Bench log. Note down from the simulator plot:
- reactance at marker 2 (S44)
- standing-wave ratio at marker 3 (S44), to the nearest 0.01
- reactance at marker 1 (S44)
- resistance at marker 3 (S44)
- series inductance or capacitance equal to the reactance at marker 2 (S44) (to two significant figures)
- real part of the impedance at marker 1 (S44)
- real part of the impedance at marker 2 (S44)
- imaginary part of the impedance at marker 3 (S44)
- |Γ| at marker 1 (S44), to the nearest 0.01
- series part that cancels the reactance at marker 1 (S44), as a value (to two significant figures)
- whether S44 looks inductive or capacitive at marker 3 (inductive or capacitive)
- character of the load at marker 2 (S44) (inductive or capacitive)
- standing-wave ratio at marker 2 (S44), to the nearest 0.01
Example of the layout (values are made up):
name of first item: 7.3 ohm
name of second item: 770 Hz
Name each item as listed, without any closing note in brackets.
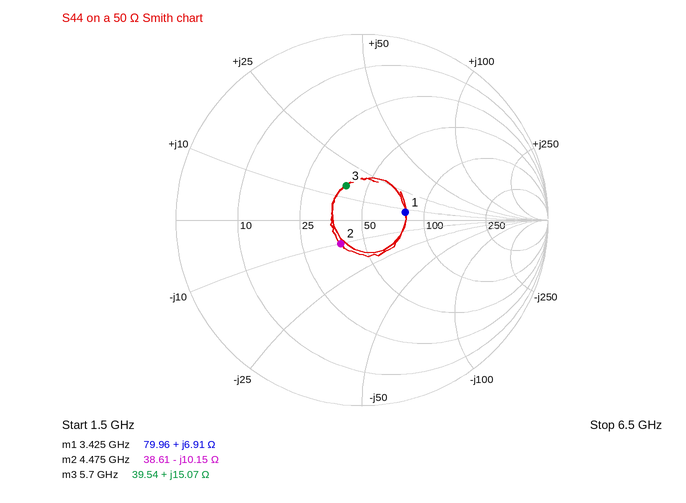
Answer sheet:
reactance at marker 2: -10.15 Ω
standing-wave ratio at marker 3 (S44), to the nearest 0.01: 1.51
reactance at marker 1: +6.91 Ω
resistance at marker 3: 39.54 Ω
series inductance or capacitance equal to the reactance at marker 2 (S44): 3.5 pF
real part of the impedance at marker 1: 79.96 Ω
real part of the impedance at marker 2: 38.61 Ω
imaginary part of the impedance at marker 3: +15.07 Ω
|Γ| at marker 1 (S44), to the nearest 0.01: 0.24
series part that cancels the reactance at marker 1 (S44), as a value: 6.7 pF
whether S44 looks inductive or capacitive at marker 3: inductive
character of the load at marker 2 (S44): capacitive
standing-wave ratio at marker 2 (S44), to the nearest 0.01: 1.41
